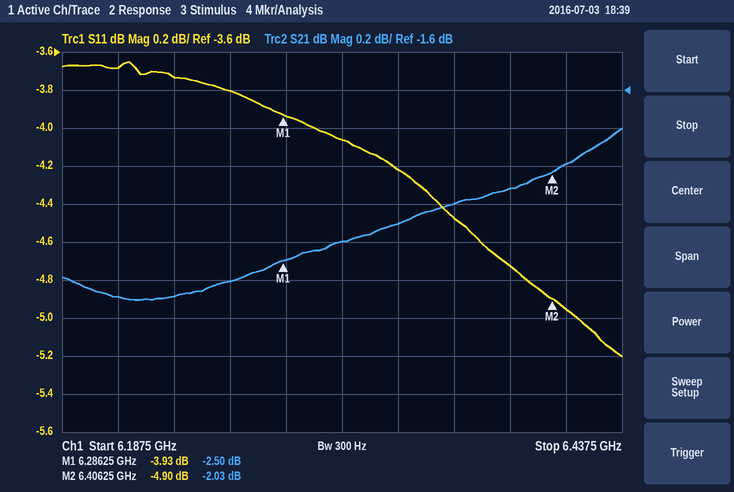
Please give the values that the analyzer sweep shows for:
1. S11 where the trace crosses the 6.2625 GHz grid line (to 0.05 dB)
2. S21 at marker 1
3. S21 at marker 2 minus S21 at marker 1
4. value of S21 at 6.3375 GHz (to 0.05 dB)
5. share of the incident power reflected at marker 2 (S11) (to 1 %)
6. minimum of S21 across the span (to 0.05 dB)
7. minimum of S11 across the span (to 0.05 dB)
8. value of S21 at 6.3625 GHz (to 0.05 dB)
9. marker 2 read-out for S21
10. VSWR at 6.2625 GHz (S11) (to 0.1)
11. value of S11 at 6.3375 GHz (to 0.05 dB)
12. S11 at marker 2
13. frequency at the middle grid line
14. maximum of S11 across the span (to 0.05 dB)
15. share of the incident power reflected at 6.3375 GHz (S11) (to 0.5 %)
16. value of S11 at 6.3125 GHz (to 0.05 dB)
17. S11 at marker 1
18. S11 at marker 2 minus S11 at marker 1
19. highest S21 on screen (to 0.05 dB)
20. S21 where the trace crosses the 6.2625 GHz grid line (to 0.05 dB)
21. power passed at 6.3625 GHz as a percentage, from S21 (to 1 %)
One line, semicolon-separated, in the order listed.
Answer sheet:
-3.80 dB; -2.50 dB; 0.47 dB; -2.30 dB; 32 %; -2.70 dB; -5.20 dB; -2.20 dB; -2.03 dB; 4.6; -4.20 dB; -4.90 dB; 6.3125 GHz; -3.65 dB; 38.0 %; -4.05 dB; -3.93 dB; -0.97 dB; -1.80 dB; -2.60 dB; 60 %
